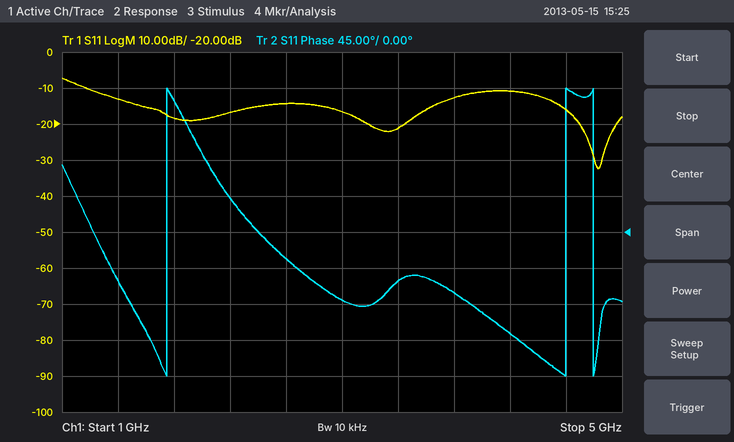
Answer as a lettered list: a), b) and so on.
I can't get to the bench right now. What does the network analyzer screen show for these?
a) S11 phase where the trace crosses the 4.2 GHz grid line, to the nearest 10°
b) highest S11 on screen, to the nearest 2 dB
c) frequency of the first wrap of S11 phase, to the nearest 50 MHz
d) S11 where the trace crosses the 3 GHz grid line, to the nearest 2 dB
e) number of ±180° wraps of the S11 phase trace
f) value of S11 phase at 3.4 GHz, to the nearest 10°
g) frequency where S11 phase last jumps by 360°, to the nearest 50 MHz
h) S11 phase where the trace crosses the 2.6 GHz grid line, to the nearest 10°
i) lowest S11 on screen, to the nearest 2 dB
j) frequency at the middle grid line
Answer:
a) -130°
b) -8 dB
c) 1.75 GHz
d) -16 dB
e) 3
f) -60°
g) 4.80 GHz
h) -30°
i) -32 dB
j) 3 GHz
